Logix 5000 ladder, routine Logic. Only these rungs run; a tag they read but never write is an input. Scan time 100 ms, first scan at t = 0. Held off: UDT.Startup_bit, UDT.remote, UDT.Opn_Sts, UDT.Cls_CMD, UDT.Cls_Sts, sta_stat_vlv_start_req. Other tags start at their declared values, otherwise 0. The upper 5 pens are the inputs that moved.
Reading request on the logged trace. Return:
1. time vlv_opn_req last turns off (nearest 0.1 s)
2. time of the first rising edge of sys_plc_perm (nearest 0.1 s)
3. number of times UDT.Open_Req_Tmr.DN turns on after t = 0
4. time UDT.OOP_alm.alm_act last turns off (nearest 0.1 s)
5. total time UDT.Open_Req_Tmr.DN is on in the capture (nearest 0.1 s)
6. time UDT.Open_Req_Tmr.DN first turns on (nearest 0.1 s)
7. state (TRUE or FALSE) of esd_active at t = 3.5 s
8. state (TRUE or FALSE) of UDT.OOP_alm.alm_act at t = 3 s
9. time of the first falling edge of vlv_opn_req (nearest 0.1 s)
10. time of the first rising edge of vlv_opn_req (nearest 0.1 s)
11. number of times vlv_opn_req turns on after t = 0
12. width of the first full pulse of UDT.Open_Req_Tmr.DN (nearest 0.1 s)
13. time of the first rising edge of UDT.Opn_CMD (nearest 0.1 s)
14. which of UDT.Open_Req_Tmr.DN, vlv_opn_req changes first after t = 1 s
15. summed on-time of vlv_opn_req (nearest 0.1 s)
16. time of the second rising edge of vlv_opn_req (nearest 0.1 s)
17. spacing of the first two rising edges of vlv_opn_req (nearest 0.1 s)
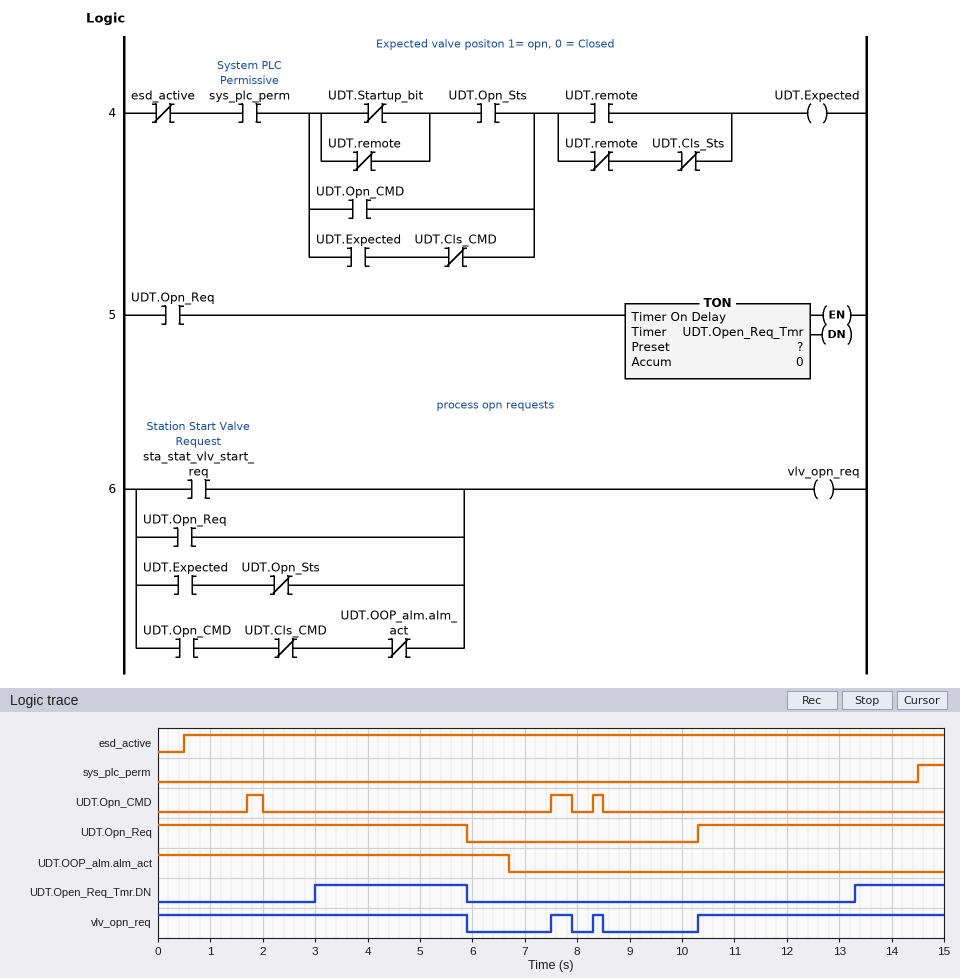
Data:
8.5 s
14.5 s
2
6.7 s
4.6 s
3.0 s
TRUE
TRUE
5.9 s
7.5 s
3
2.9 s
1.7 s
UDT.Open_Req_Tmr.DN
11.2 s
8.3 s
0.8 s
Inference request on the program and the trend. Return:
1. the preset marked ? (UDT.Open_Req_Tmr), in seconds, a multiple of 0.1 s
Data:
3.0 s
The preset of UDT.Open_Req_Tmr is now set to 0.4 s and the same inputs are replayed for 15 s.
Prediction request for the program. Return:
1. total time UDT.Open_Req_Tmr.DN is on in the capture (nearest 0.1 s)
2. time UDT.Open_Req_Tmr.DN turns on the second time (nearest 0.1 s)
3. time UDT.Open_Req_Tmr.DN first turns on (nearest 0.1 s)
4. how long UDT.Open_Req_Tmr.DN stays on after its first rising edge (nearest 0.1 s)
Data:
9.8 s
10.7 s
0.4 s
5.5 s
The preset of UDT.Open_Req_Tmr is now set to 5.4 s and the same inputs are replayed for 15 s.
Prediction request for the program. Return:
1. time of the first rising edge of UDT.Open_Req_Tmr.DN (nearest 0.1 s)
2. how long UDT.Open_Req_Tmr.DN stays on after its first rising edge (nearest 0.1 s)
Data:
5.4 s
0.5 s
